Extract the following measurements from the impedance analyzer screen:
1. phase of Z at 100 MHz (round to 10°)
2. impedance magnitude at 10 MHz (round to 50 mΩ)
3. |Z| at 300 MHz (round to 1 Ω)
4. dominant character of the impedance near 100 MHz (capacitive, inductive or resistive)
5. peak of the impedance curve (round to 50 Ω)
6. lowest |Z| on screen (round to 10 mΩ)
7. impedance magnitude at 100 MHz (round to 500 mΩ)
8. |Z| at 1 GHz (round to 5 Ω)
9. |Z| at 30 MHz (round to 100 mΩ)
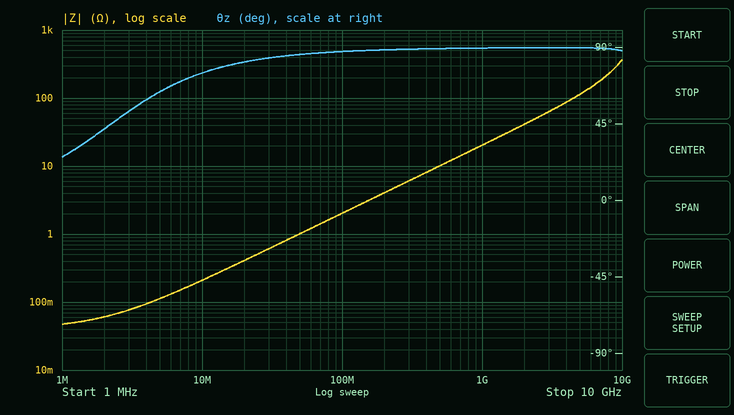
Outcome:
90°
200 mΩ
6 Ω
inductive
350 Ω
50 mΩ
2.0 Ω
20 Ω
600 mΩ
